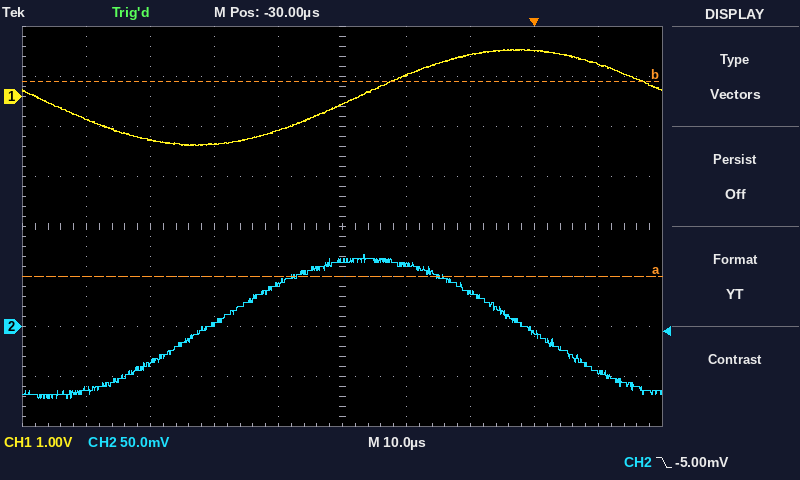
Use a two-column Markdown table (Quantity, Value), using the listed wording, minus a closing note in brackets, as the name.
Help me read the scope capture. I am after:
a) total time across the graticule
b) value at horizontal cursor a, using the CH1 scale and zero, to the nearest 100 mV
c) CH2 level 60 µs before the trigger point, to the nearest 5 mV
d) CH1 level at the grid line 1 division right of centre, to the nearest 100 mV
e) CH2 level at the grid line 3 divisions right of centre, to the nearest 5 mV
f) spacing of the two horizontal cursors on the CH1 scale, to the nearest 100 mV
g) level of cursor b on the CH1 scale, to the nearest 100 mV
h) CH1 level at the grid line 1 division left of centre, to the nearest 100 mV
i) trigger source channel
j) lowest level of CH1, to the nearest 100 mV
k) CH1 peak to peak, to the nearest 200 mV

| Quantity | Value |
|---|---|
| total time across the graticule | 100 µs |
| value at horizontal cursor a, using the CH1 scale and zero, to the nearest 100 mV | -3.6 V |
| CH2 level 60 µs before the trigger point, to the nearest 5 mV | -35 mV |
| CH1 level at the grid line 1 division right of centre, to the nearest 100 mV | 400 mV |
| CH2 level at the grid line 3 divisions right of centre, to the nearest 5 mV | -5 mV |
| spacing of the two horizontal cursors on the CH1 scale, to the nearest 100 mV | 3.9 V |
| level of cursor b on the CH1 scale, to the nearest 100 mV | 300 mV |
| CH1 level at the grid line 1 division left of centre, to the nearest 100 mV | -700 mV |
| trigger source channel | CH2 |
| lowest level of CH1, to the nearest 100 mV | -1.0 V |
| CH1 peak to peak, to the nearest 200 mV | 2.0 V |
